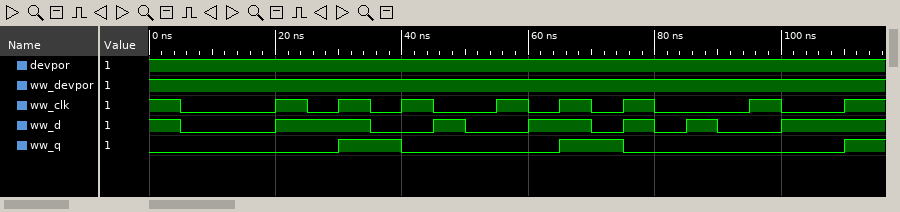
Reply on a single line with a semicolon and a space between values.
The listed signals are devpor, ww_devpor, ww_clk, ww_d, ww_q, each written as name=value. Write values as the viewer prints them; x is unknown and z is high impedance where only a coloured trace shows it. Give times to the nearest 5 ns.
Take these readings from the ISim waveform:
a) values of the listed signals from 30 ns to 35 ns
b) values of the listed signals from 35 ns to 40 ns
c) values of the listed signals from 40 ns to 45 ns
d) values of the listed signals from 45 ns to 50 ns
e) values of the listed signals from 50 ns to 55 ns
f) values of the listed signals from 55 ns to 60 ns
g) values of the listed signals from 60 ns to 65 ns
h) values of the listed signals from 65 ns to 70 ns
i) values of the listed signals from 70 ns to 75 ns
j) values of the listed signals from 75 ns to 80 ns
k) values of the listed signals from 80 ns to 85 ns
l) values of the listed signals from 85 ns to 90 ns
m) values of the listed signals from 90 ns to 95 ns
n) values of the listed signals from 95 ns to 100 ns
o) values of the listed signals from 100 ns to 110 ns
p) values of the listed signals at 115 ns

devpor=1, ww_devpor=1, ww_clk=1, ww_d=1, ww_q=1; devpor=1, ww_devpor=1, ww_clk=0, ww_d=0, ww_q=1; devpor=1, ww_devpor=1, ww_clk=1, ww_d=0, ww_q=0; devpor=1, ww_devpor=1, ww_clk=0, ww_d=1, ww_q=0; devpor=1, ww_devpor=1, ww_clk=0, ww_d=0, ww_q=0; devpor=1, ww_devpor=1, ww_clk=1, ww_d=0, ww_q=0; devpor=1, ww_devpor=1, ww_clk=0, ww_d=1, ww_q=0; devpor=1, ww_devpor=1, ww_clk=1, ww_d=1, ww_q=1; devpor=1, ww_devpor=1, ww_clk=0, ww_d=0, ww_q=1; devpor=1, ww_devpor=1, ww_clk=1, ww_d=1, ww_q=0; devpor=1, ww_devpor=1, ww_clk=0, ww_d=0, ww_q=0; devpor=1, ww_devpor=1, ww_clk=0, ww_d=1, ww_q=0; devpor=1, ww_devpor=1, ww_clk=0, ww_d=0, ww_q=0; devpor=1, ww_devpor=1, ww_clk=1, ww_d=0, ww_q=0; devpor=1, ww_devpor=1, ww_clk=0, ww_d=1, ww_q=0; devpor=1, ww_devpor=1, ww_clk=1, ww_d=1, ww_q=1
